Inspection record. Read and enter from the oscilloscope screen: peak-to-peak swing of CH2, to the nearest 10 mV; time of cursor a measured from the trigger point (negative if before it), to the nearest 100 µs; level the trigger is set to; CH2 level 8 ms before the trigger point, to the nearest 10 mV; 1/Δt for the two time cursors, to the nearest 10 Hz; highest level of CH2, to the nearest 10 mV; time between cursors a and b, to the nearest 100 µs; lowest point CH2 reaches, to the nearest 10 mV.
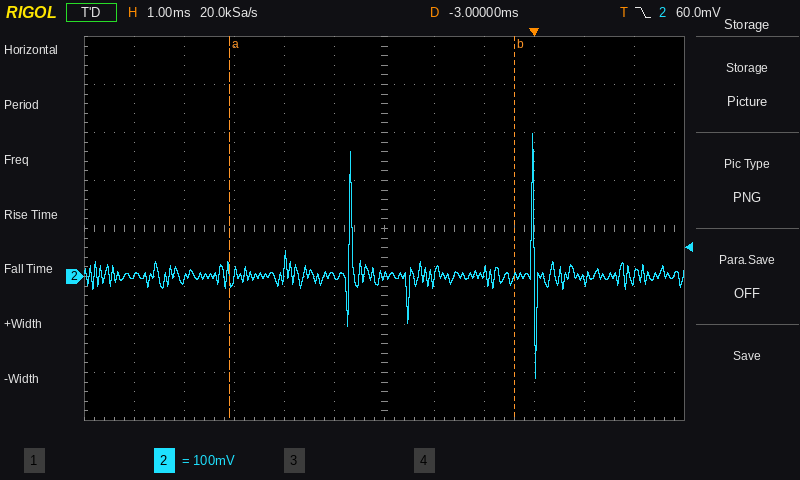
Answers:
510 mV
-6.1 ms
60.0 mV
0 mV
180 Hz
300 mV
5.7 ms
-210 mV
